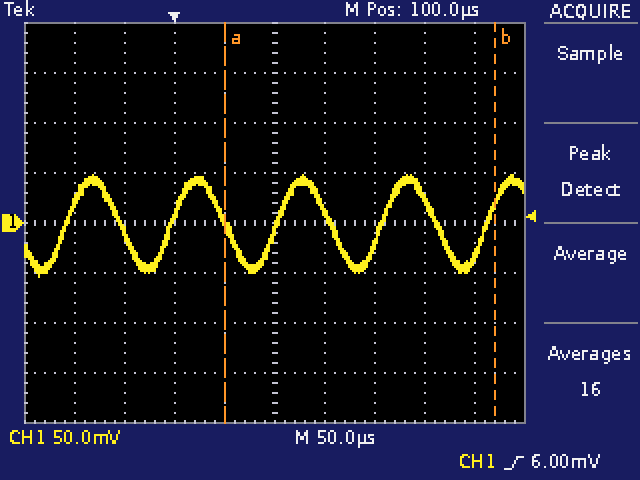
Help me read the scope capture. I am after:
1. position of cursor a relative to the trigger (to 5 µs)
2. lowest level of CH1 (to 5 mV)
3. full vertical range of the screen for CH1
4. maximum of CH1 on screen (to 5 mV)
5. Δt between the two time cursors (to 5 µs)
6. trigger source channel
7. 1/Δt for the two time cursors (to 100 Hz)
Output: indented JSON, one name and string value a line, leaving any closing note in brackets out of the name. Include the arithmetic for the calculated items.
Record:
{
  "position of cursor a relative to the trigger": "+50 µs",
  "lowest level of CH1": "-55 mV",
  "full vertical range of the screen for CH1": "400 mV",
  "maximum of CH1 on screen": "50 mV",
  "Δt between the two time cursors": "270 µs",
  "trigger source channel": "CH1",
  "1/Δt for the two time cursors": "1 / 270 µs ≈ 3.7 kHz"
}
